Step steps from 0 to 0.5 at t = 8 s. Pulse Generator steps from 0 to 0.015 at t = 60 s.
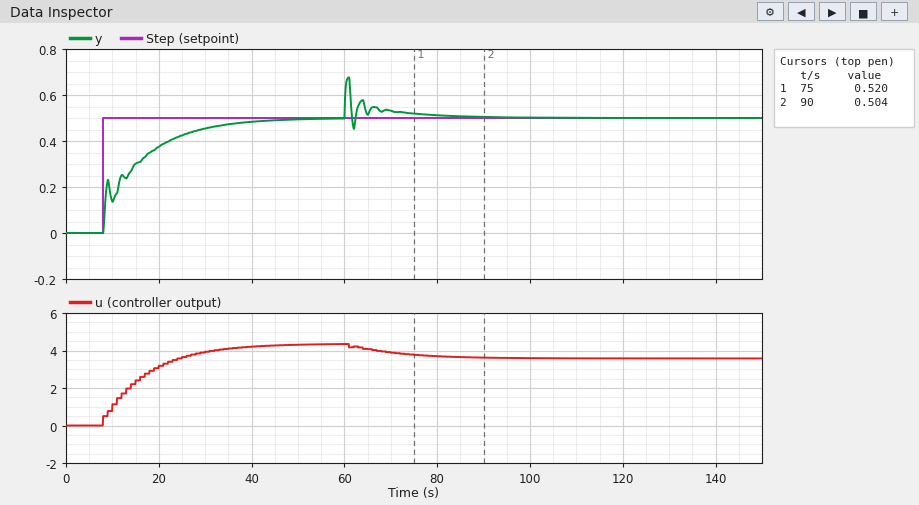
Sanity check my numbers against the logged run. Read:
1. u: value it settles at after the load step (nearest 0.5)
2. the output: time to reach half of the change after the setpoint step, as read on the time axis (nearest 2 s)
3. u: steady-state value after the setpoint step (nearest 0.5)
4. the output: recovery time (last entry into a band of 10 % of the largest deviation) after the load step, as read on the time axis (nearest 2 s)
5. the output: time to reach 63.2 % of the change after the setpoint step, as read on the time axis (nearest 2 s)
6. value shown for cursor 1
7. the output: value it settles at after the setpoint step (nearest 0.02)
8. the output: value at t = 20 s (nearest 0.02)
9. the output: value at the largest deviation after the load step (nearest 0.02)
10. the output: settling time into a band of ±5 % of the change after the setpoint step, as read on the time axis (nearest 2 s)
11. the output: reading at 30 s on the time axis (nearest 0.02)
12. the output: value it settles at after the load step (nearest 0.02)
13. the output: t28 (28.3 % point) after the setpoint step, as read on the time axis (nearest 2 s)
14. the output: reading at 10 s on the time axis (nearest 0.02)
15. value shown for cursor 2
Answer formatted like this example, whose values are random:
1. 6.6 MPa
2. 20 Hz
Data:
1. 3.5
2. 12 s
3. 4.5
4. 76 s
5. 16 s
6. 0.520
7. 0.50
8. 0.38
9. 0.68
10. 36 s
11. 0.46
12. 0.50
13. 8 s
14. 0.14
15. 0.504
